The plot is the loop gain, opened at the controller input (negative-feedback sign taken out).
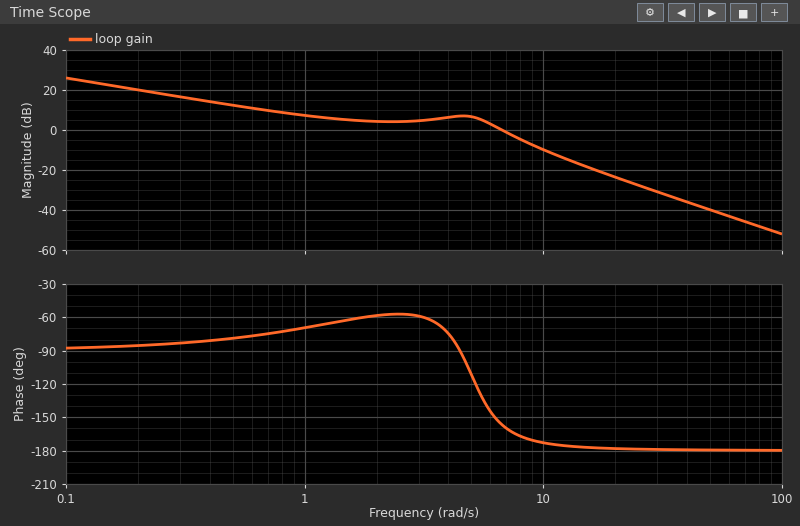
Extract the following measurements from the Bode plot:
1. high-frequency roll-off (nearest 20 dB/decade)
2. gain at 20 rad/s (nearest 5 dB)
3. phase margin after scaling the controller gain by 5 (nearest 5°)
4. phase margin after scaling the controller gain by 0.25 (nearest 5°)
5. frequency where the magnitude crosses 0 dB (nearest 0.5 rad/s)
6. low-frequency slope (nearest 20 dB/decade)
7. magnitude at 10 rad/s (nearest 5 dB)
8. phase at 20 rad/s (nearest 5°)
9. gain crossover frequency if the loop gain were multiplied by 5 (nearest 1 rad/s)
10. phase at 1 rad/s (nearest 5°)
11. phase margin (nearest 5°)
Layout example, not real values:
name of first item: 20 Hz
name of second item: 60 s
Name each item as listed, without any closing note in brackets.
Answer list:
high-frequency roll-off: -40 dB/decade
gain at 20 rad/s: -25 dB
phase margin after scaling the controller gain by 5: 5°
phase margin after scaling the controller gain by 0.25: 100°
frequency where the magnitude crosses 0 dB: 6.5 rad/s
low-frequency slope: -20 dB/decade
magnitude at 10 rad/s: -10 dB
phase at 20 rad/s: -180°
gain crossover frequency if the loop gain were multiplied by 5: 12 rad/s
phase at 1 rad/s: -70°
phase margin: 25°
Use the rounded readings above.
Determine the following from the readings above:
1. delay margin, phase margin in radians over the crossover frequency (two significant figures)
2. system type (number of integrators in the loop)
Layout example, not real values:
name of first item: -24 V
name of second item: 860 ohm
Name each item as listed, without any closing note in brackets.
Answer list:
delay margin, phase margin in radians over the crossover frequency: 0.067 s
system type: 1
